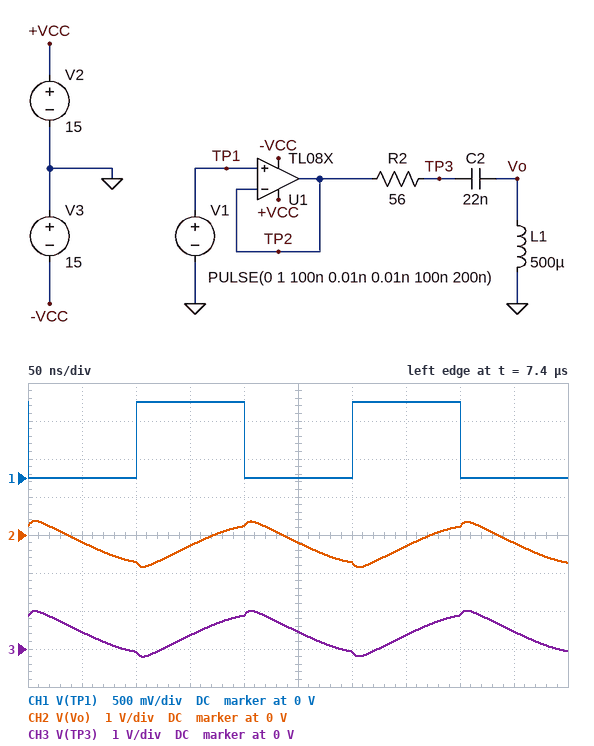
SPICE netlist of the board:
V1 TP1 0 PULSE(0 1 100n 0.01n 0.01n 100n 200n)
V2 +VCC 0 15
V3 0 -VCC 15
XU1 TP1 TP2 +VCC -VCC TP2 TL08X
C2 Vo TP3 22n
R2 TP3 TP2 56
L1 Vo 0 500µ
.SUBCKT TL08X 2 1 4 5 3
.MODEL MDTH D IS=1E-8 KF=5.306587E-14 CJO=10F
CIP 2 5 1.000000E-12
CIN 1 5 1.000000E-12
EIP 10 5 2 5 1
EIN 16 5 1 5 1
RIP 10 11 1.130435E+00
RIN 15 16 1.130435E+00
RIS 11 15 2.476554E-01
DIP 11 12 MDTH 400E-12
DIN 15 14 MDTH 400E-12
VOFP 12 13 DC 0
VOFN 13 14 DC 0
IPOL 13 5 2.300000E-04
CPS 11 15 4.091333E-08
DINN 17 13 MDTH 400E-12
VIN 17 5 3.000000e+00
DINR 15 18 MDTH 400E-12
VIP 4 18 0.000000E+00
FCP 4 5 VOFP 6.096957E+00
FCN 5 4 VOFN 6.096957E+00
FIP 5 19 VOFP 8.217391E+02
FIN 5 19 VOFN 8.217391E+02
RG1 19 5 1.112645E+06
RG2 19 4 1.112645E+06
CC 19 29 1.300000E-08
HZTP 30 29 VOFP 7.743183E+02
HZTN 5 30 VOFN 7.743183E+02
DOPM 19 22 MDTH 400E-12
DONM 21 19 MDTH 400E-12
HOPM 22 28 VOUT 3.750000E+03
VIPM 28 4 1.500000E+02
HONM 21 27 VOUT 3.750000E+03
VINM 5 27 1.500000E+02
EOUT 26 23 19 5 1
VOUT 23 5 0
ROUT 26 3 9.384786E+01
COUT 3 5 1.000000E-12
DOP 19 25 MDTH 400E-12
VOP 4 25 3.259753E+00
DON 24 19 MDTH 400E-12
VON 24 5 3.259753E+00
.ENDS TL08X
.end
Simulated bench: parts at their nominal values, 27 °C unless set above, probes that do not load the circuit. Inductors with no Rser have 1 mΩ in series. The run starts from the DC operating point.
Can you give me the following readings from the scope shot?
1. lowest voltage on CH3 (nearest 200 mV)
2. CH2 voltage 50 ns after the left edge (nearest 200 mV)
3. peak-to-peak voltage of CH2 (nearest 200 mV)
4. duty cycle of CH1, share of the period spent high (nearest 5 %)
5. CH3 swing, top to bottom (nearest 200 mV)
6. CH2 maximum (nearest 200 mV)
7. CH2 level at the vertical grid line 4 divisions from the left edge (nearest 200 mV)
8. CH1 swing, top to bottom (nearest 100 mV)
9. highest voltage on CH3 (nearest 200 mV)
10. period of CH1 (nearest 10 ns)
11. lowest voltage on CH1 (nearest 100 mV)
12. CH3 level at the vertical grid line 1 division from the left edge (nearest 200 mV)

-200 mV
-200 mV
1.2 V
50 %
1.2 V
400 mV
200 mV
1.0 V
1.0 V
200 ns
0 V
400 mV
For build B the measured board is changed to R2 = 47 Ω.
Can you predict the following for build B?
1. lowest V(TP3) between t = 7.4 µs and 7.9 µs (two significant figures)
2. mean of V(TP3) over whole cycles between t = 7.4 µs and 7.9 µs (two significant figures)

-190 mV
410 mV
